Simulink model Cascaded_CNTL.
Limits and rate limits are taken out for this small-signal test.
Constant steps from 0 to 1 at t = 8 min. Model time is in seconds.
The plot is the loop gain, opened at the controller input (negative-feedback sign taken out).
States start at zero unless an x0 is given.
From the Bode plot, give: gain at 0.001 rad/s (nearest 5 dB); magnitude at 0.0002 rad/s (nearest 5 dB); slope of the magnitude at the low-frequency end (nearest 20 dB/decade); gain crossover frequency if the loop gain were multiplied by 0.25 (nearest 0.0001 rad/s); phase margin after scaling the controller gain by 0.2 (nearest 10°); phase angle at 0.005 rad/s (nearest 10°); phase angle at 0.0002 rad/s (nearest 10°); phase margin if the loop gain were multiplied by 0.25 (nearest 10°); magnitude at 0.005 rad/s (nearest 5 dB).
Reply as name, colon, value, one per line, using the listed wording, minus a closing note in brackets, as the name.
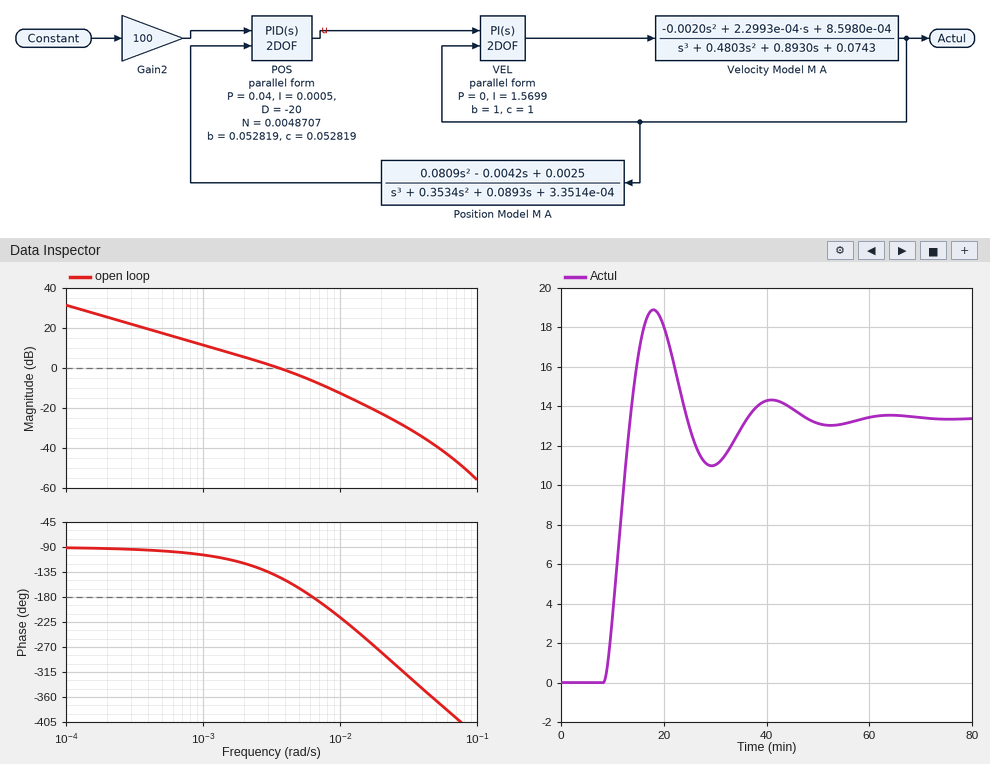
gain at 0.001 rad/s: 10 dB
magnitude at 0.0002 rad/s: 25 dB
slope of the magnitude at the low-frequency end: -20 dB/decade
gain crossover frequency if the loop gain were multiplied by 0.25: 0.0009 rad/s
phase margin after scaling the controller gain by 0.2: 80°
phase angle at 0.005 rad/s: -160°
phase angle at 0.0002 rad/s: -90°
phase margin if the loop gain were multiplied by 0.25: 80°
magnitude at 0.005 rad/s: -5 dB
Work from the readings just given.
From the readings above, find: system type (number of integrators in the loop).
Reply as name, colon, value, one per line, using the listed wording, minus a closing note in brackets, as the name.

system type: 1
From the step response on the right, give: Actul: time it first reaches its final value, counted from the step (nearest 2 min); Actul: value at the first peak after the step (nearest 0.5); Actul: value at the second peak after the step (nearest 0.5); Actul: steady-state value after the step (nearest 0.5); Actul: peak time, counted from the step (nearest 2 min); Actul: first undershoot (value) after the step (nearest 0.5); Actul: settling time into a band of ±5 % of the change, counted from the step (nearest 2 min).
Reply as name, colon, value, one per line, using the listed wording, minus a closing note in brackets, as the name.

Actul: time it first reaches its final value, counted from the step: 6 min
Actul: value at the first peak after the step: 19.0
Actul: value at the second peak after the step: 14.5
Actul: steady-state value after the step: 13.5
Actul: peak time, counted from the step: 10 min
Actul: first undershoot (value) after the step: 11.0
Actul: settling time into a band of ±5 % of the change, counted from the step: 36 min
